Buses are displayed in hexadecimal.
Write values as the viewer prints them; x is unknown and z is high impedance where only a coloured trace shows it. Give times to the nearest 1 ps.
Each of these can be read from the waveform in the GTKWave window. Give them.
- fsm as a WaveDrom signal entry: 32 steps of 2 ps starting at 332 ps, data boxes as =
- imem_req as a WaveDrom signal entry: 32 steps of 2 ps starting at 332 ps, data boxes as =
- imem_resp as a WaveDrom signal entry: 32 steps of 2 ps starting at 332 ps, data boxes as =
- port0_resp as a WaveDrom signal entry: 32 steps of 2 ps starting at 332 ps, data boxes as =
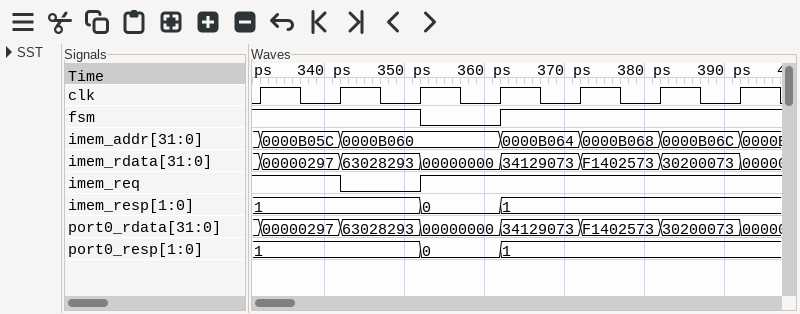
{name: 'fsm', wave: '1.........0....1................'}
{name: 'imem_req', wave: '1....0....1.....................'}
{name: 'imem_resp', wave: '=.........=....=................', data: '1 0 1'}
{name: 'port0_resp', wave: '=.........=....=................', data: '1 0 1'}
